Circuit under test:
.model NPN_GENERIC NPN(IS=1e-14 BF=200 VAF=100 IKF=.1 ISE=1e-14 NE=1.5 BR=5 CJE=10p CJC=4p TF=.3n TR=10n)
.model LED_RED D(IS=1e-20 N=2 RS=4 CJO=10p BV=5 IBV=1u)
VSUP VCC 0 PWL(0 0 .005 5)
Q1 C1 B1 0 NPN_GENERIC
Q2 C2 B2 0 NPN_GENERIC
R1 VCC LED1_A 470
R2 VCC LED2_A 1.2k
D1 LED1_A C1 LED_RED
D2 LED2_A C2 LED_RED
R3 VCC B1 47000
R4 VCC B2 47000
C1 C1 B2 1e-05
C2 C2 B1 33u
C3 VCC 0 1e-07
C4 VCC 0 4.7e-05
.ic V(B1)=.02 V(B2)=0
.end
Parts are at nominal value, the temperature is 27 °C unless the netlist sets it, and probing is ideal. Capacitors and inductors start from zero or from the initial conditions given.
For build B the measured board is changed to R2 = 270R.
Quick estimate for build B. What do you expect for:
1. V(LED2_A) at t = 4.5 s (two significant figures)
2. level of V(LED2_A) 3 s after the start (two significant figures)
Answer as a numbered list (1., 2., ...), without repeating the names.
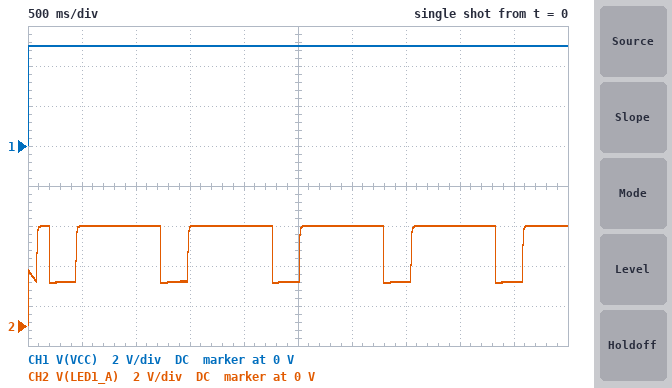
1. 5.0 V
2. 2.3 V
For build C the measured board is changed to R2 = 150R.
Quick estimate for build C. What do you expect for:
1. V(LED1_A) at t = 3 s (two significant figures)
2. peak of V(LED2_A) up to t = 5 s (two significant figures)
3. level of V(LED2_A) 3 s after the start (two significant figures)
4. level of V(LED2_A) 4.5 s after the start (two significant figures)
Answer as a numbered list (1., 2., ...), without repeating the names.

1. 2.2 V
2. 5.0 V
3. 5.0 V
4. 2.7 V
